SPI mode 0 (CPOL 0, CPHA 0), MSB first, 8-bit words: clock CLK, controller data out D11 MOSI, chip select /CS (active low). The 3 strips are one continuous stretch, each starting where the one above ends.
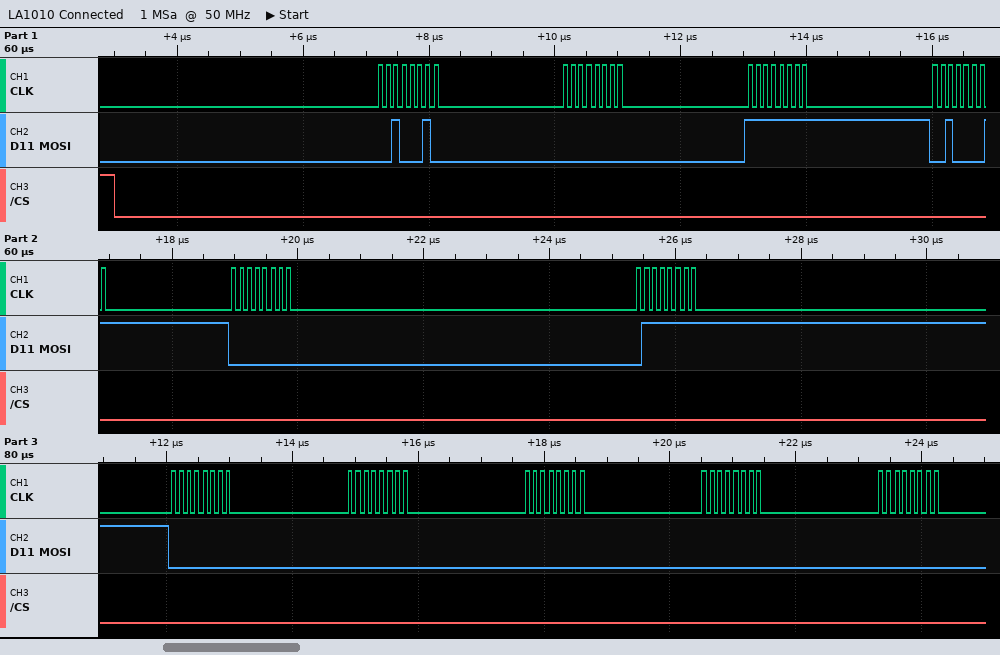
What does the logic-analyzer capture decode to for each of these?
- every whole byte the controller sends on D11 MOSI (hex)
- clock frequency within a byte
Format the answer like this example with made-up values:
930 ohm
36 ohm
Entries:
22 00 FF 21 00 7F 00 00 00 00 00
8 MHz
